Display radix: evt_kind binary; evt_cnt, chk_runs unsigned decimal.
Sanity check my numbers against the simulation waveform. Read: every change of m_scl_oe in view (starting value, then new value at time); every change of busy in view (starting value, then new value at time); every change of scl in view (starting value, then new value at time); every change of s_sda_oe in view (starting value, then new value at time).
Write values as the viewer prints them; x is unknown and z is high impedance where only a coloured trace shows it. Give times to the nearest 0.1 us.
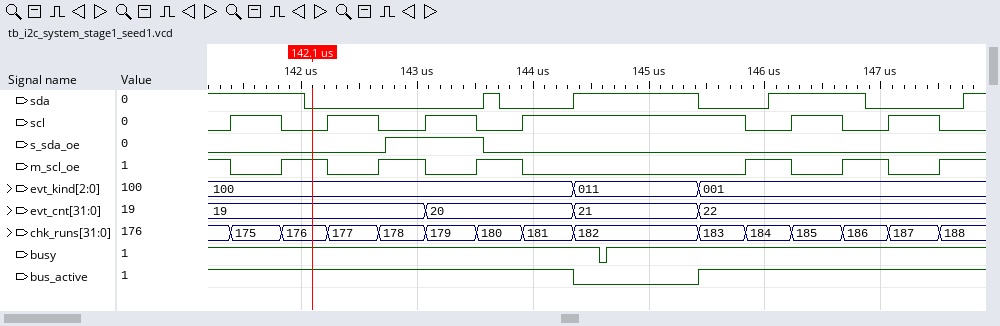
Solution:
1, 0 at 141.4 us, 1 at 141.8 us, 0 at 142.2 us, 1 at 142.7 us, 0 at 143.1 us, 1 at 143.5 us, 0 at 143.9 us, 1 at 145.8 us, 0 at 146.2 us, 1 at 146.7 us, 0 at 147.1 us, 1 at 147.5 us
1, 0 at 144.6 us, 1 at 144.6 us
0, 1 at 141.4 us, 0 at 141.8 us, 1 at 142.2 us, 0 at 142.7 us, 1 at 143.1 us, 0 at 143.5 us, 1 at 143.9 us, 0 at 145.8 us, 1 at 146.2 us, 0 at 146.7 us, 1 at 147.1 us, 0 at 147.5 us
0, 1 at 142.7 us, 0 at 143.6 us
